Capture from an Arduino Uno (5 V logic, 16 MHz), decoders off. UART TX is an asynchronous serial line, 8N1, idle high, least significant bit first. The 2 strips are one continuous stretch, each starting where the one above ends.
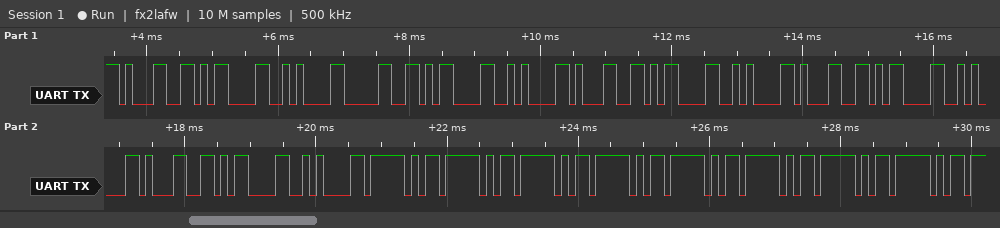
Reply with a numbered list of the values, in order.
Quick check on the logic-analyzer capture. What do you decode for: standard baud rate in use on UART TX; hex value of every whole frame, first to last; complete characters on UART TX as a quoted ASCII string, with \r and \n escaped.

1. 9600 baud
2. 31 0D 0A 30 0D 0A 31 0D 0A 31 0D 0A 31 0D 0A 5F 5F 5F 5F 5F 5F 5F 5F
3. "1\r\n0\r\n1\r\n1\r\n1\r\n________"
